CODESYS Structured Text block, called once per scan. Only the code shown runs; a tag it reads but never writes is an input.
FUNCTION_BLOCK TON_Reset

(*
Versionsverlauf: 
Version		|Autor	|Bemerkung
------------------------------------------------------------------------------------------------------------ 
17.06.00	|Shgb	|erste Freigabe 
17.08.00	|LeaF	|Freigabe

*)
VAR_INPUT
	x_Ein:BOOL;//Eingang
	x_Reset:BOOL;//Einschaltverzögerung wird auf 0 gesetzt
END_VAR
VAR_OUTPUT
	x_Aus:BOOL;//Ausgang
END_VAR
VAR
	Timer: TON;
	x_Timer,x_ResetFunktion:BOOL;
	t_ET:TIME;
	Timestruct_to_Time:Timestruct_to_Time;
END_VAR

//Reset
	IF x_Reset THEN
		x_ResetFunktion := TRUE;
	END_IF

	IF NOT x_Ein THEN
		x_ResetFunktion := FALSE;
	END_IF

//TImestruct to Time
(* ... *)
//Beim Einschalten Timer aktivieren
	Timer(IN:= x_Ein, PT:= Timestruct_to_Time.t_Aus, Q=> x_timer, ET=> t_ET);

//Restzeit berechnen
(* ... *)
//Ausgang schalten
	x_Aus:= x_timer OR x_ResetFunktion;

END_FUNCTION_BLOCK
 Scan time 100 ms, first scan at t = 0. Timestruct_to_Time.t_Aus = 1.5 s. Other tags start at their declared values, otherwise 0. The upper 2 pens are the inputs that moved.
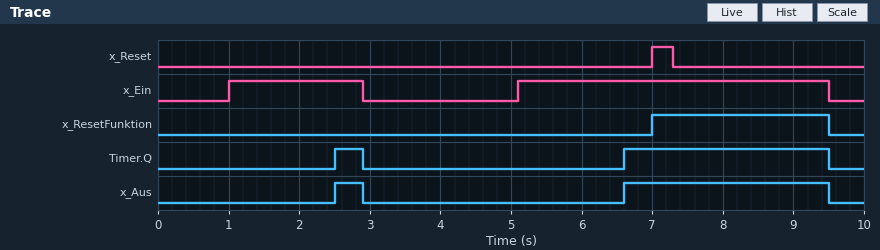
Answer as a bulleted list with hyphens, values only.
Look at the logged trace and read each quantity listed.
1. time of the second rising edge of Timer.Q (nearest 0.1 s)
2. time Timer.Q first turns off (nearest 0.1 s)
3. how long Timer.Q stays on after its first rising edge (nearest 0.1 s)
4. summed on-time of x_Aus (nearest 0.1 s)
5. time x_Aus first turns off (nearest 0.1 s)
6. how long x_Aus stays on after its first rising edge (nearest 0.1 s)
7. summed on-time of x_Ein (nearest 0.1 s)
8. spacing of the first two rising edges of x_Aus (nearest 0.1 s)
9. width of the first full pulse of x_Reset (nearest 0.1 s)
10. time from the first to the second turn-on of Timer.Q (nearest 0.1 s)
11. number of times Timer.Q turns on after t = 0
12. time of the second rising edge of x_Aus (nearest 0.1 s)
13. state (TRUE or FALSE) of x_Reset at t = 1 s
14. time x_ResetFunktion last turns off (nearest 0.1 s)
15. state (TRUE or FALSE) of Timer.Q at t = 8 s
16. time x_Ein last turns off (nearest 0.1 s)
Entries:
- 6.6 s
- 2.9 s
- 0.4 s
- 3.3 s
- 2.9 s
- 0.4 s
- 6.3 s
- 4.1 s
- 0.3 s
- 4.1 s
- 2
- 6.6 s
- FALSE
- 9.5 s
- TRUE
- 9.5 s
